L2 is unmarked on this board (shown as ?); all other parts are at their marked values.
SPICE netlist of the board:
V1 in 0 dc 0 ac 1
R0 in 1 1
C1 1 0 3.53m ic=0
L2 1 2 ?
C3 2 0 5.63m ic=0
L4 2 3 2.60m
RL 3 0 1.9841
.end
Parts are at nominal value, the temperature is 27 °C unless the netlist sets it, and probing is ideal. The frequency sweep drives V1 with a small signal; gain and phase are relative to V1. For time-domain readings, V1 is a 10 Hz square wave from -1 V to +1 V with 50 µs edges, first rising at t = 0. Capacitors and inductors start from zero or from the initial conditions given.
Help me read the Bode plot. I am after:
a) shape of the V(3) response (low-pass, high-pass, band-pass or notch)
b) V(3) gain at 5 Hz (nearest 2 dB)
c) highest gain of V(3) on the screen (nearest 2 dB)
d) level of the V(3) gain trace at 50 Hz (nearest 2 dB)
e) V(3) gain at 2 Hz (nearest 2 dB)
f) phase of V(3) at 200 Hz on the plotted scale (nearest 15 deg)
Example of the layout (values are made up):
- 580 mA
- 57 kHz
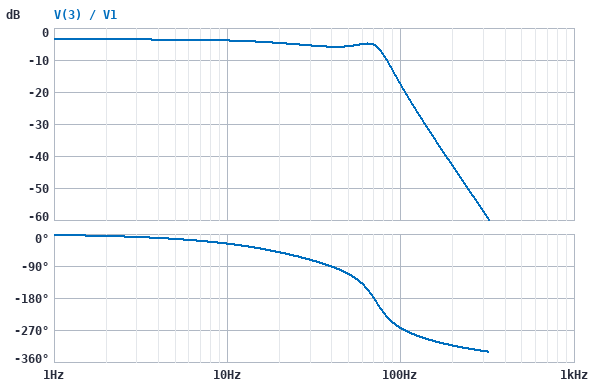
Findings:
- low-pass
- -4 dB
- -4 dB
- -6 dB
- -4 dB
- -315 deg
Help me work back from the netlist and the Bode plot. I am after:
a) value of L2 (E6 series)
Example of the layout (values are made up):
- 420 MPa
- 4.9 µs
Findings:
- 2.2 mH
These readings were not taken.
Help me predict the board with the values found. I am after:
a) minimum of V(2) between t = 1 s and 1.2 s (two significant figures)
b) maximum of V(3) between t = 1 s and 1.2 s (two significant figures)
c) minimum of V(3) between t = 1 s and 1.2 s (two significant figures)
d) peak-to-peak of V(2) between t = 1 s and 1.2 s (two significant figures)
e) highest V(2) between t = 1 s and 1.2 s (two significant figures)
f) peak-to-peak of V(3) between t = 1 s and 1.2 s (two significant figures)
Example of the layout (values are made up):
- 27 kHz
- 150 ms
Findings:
- -710 mV
- 700 mV
- -700 mV
- 1.4 V
- 710 mV
- 1.4 V
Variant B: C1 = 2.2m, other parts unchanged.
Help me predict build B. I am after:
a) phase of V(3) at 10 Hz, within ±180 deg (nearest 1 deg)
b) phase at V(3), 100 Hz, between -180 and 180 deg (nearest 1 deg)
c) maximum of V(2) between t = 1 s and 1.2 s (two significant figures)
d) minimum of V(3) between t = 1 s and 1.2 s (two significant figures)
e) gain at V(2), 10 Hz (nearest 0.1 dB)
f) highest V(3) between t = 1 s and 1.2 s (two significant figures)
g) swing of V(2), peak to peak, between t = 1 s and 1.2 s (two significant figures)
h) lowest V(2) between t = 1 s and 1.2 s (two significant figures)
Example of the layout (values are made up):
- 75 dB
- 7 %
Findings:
- -24 deg
- 123 deg
- 680 mV
- -670 mV
- -3.7 dB
- 670 mV
- 1.4 V
- -680 mV
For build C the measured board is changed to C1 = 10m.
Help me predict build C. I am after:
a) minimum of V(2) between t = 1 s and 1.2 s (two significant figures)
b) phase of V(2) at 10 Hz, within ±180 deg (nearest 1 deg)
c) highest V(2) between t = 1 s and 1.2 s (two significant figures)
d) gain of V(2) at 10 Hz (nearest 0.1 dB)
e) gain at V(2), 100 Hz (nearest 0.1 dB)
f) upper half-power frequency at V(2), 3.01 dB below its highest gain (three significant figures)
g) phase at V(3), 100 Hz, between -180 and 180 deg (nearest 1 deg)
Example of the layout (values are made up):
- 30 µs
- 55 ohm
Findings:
- -700 mV
- -35 deg
- 700 mV
- -4.7 dB
- -25.8 dB
- 63.1 Hz
- 68 deg
